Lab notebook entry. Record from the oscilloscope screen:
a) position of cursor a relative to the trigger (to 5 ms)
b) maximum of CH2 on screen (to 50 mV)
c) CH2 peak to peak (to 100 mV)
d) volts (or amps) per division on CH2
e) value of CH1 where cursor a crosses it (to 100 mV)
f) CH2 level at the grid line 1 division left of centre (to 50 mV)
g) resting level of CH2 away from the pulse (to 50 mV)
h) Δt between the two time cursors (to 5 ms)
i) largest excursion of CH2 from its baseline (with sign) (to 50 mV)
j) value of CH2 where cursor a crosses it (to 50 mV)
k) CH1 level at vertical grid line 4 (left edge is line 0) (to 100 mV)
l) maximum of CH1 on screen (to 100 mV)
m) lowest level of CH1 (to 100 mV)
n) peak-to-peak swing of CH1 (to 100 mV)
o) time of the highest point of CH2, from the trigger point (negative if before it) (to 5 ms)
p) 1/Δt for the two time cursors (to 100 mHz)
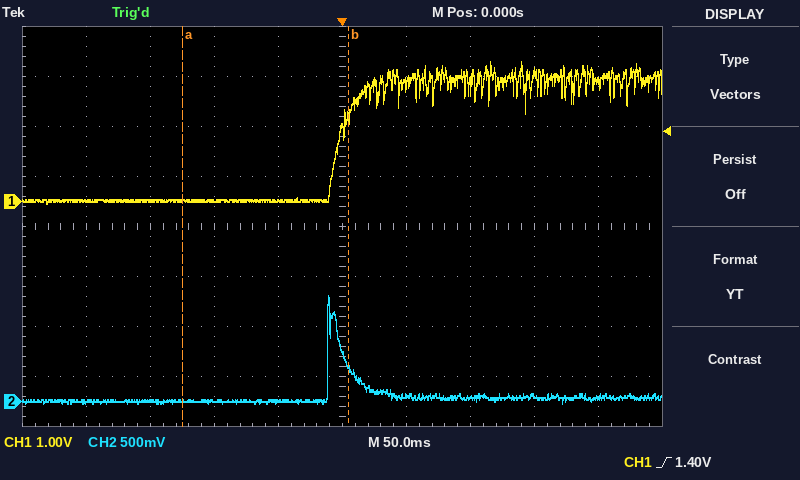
-125 ms
1.05 V
1.10 V
500 mV
0.0 V
0 mV
0 mV
130 ms
+1.05 V
0 mV
0.0 V
2.8 V
0.0 V
2.8 V
-10 ms
7.7 Hz
